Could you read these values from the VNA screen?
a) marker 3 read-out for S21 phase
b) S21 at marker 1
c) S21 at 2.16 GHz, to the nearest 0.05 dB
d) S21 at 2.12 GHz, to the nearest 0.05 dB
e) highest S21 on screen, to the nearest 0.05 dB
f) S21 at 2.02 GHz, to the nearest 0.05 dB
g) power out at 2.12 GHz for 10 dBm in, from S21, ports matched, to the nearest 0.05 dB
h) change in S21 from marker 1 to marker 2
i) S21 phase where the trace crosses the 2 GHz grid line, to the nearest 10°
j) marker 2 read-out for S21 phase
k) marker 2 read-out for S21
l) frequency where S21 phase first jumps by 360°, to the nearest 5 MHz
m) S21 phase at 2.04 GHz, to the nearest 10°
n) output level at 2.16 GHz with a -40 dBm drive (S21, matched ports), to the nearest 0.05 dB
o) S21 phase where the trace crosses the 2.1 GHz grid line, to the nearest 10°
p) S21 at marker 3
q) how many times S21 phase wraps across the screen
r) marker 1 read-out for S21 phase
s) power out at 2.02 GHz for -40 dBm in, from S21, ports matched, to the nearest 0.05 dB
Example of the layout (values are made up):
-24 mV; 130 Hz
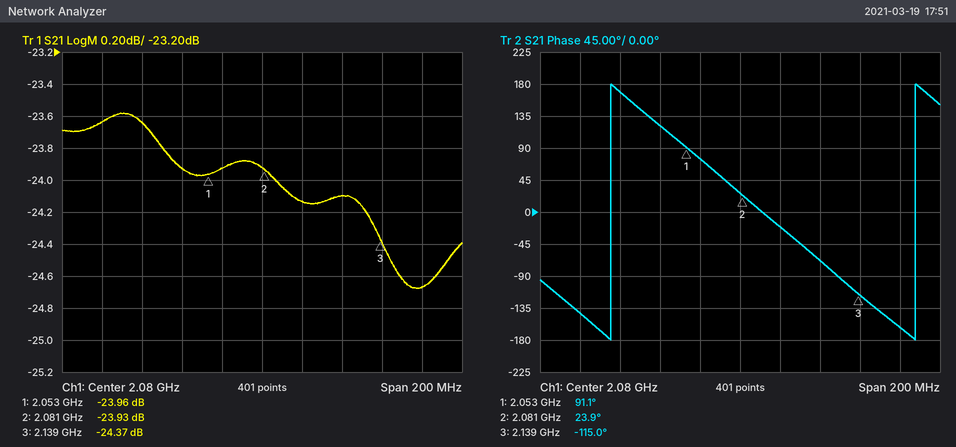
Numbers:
-115.0°; -23.96 dB; -24.65 dB; -24.10 dB; -23.60 dB; -23.65 dB; -14.10 dBm; 0.03 dB; -140°; 23.9°; -23.93 dB; 2.015 GHz; 120°; -64.65 dBm; -20°; -24.37 dB; 2; 91.1°; -63.65 dBm
